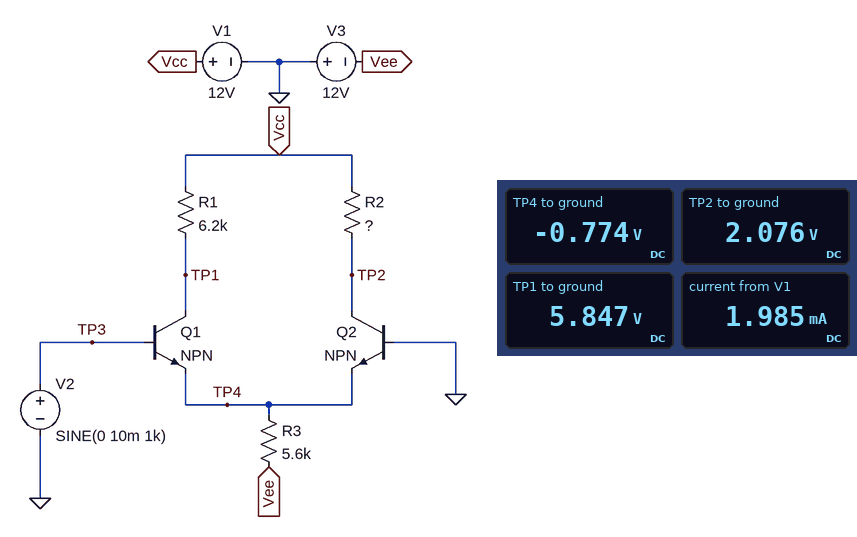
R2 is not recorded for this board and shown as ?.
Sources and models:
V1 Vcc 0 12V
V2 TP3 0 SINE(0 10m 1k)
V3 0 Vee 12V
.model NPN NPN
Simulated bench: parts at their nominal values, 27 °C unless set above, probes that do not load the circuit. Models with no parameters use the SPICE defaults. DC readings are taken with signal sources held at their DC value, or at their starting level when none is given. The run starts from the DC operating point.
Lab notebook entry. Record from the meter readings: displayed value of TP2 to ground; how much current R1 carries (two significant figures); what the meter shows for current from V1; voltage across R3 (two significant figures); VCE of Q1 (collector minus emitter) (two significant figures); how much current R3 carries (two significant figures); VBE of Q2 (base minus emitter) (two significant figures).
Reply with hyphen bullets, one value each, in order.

- 2.076 V
- 990 µA
- 1.985 mA
- 11 V
- 6.6 V
- 2.0 mA
- 770 mV
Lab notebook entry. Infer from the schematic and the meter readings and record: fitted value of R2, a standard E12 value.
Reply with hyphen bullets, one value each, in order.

- 10 kΩ
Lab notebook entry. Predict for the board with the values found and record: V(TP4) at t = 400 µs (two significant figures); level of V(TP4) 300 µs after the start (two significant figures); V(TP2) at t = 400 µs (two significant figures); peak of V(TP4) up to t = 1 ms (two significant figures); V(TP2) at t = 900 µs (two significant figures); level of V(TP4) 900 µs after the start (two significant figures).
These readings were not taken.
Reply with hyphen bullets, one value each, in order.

- -770 mV
- -770 mV
- 3.2 V
- -770 mV
- 960 mV
- -780 mV
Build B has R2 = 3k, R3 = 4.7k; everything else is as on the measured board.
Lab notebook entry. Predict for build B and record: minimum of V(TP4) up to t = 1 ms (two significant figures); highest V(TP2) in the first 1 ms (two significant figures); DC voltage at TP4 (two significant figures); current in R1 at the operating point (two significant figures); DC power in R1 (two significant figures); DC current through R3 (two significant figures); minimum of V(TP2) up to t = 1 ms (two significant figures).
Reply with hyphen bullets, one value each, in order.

- -780 mV
- 9.1 V
- -780 mV
- 1.2 mA
- 8.7 mW
- 2.4 mA
- 7.8 V
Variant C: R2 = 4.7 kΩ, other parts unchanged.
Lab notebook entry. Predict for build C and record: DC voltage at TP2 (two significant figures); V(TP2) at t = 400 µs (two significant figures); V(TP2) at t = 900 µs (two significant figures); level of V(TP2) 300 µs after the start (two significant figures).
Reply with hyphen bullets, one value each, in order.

- 7.3 V
- 7.9 V
- 6.8 V
- 8.2 V
